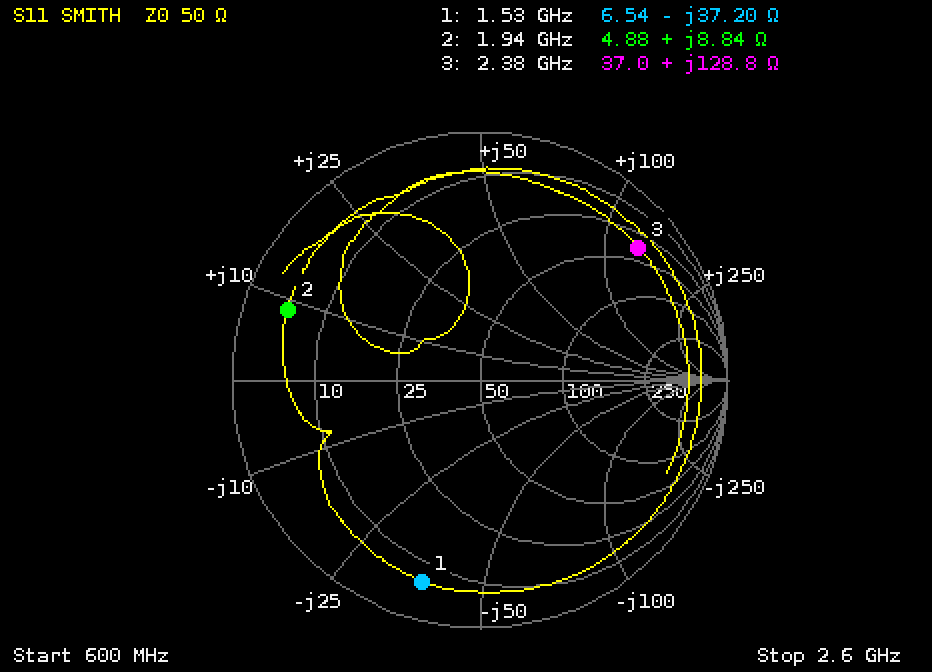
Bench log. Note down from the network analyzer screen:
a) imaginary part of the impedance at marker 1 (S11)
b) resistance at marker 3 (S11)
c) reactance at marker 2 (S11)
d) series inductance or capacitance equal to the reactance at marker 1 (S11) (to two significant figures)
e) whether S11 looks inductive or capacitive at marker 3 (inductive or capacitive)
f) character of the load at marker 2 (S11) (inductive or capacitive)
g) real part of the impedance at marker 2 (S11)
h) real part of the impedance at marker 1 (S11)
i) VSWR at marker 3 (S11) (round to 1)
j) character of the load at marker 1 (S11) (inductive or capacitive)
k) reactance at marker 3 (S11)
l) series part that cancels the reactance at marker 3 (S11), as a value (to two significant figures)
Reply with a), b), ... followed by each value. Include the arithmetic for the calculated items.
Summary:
a) -37.20 Ω
b) 37.0 Ω
c) +8.84 Ω
d) C = 1/(2π × 1.53 GHz × 37.2 Ω) ≈ 2.8 pF
e) inductive
f) inductive
g) 4.88 Ω
h) 6.54 Ω
i) 11
j) capacitive
k) +128.8 Ω
l) C = 1/(2π × 2.38 GHz × 128.8 Ω) ≈ 519 fF, so 520 fF to two significant figures
